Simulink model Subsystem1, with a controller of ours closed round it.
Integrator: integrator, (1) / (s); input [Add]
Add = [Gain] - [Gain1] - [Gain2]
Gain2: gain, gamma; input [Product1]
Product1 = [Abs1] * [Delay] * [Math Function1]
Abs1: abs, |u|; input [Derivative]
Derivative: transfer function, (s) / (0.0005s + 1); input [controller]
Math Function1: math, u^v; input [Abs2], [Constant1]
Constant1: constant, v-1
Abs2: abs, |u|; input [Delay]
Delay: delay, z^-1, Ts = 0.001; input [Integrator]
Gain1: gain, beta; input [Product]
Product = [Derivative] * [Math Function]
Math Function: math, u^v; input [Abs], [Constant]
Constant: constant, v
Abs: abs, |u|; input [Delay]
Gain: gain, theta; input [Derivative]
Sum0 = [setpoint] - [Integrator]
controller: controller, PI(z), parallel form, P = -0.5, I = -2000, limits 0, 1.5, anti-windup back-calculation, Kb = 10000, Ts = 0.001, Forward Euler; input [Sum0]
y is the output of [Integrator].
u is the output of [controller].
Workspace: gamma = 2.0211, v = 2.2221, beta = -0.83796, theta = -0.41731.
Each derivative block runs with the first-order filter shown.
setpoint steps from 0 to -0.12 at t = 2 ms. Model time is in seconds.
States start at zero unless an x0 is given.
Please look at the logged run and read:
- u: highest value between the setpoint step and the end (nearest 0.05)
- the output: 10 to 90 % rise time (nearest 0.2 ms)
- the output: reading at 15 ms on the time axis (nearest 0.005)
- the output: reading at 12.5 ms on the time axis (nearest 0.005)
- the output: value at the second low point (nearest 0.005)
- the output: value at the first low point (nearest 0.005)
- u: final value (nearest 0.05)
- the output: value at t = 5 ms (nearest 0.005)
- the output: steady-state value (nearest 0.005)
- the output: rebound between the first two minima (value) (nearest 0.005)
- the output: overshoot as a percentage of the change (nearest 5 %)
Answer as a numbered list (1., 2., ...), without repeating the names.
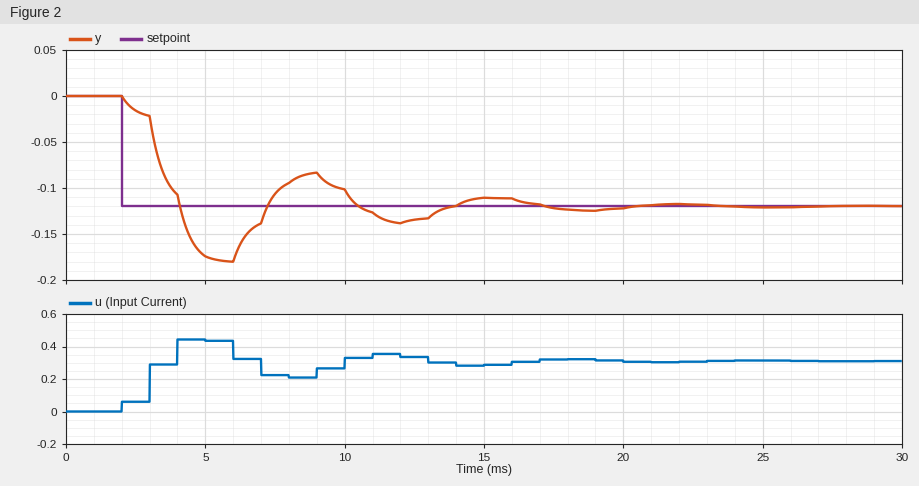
1. 0.45
2. 1.6 ms
3. -0.110
4. -0.135
5. -0.140
6. -0.180
7. 0.30
8. -0.175
9. -0.120
10. -0.085
11. 50 %
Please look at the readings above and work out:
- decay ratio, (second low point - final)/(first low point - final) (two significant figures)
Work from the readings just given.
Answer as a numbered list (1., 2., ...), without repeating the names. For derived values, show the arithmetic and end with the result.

1. (-0.14 - (-0.12)) / (-0.18 - (-0.12)) = 0.33
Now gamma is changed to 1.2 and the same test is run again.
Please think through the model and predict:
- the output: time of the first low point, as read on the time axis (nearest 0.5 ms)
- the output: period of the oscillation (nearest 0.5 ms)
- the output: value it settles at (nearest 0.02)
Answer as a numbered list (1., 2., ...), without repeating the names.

1. 6.0 ms
2. 6.0 ms
3. -0.12
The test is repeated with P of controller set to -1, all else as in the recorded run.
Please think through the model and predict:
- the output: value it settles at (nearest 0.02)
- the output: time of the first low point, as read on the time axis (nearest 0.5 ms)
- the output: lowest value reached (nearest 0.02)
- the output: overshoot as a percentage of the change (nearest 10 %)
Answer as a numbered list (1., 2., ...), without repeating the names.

1. -0.12
2. 5.0 ms
3. -0.16
4. 30 %
